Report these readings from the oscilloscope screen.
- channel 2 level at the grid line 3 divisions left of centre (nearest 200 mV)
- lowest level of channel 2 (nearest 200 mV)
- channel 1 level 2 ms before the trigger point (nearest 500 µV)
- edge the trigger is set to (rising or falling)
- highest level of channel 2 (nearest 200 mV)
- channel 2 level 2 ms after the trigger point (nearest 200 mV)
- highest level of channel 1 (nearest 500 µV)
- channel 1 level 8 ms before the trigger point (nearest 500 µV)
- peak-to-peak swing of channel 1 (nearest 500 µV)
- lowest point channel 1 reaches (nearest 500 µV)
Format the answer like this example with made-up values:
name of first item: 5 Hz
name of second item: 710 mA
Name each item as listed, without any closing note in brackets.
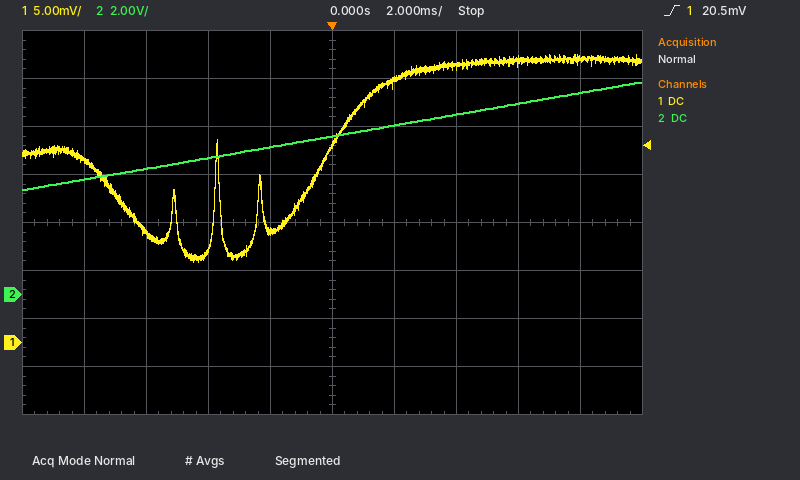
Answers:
channel 2 level at the grid line 3 divisions left of centre: 5.2 V
lowest level of channel 2: 4.4 V
channel 1 level 2 ms before the trigger point: 11.5 mV
edge the trigger is set to: rising
highest level of channel 2: 8.8 V
channel 2 level 2 ms after the trigger point: 7.0 V
highest level of channel 1: 30.0 mV
channel 1 level 8 ms before the trigger point: 19.0 mV
peak-to-peak swing of channel 1: 21.5 mV
lowest point channel 1 reaches: 8.5 mV
